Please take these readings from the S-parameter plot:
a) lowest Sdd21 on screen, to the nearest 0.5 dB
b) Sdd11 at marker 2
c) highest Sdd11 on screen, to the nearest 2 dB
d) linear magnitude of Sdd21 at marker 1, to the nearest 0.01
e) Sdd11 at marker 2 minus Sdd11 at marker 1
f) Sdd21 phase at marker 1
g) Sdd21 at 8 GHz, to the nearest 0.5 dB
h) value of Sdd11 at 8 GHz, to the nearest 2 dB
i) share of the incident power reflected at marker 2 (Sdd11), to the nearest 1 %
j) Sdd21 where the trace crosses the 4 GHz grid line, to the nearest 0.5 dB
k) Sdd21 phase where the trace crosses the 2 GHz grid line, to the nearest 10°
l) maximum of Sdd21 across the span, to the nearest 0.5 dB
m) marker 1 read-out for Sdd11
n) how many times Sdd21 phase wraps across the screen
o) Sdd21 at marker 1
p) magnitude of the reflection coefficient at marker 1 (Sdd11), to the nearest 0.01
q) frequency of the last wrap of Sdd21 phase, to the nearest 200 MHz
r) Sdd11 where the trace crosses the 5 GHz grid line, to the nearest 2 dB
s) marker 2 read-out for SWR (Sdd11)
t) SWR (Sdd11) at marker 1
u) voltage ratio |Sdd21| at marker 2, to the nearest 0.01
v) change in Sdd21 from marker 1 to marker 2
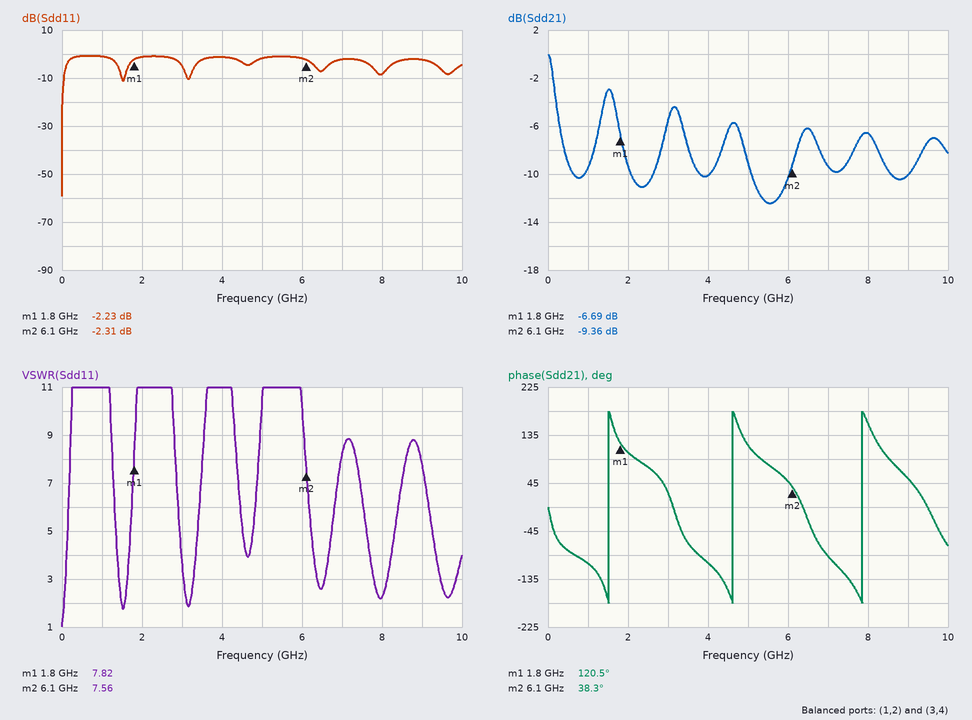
-12.5 dB
-2.31 dB
0 dB
0.46
-0.08 dB
120.5°
-6.5 dB
-8 dB
59 %
-10.0 dB
100°
0.0 dB
-2.23 dB
3
-6.69 dB
0.77
7.8 GHz
-2 dB
7.56
7.82
0.34
-2.67 dB
